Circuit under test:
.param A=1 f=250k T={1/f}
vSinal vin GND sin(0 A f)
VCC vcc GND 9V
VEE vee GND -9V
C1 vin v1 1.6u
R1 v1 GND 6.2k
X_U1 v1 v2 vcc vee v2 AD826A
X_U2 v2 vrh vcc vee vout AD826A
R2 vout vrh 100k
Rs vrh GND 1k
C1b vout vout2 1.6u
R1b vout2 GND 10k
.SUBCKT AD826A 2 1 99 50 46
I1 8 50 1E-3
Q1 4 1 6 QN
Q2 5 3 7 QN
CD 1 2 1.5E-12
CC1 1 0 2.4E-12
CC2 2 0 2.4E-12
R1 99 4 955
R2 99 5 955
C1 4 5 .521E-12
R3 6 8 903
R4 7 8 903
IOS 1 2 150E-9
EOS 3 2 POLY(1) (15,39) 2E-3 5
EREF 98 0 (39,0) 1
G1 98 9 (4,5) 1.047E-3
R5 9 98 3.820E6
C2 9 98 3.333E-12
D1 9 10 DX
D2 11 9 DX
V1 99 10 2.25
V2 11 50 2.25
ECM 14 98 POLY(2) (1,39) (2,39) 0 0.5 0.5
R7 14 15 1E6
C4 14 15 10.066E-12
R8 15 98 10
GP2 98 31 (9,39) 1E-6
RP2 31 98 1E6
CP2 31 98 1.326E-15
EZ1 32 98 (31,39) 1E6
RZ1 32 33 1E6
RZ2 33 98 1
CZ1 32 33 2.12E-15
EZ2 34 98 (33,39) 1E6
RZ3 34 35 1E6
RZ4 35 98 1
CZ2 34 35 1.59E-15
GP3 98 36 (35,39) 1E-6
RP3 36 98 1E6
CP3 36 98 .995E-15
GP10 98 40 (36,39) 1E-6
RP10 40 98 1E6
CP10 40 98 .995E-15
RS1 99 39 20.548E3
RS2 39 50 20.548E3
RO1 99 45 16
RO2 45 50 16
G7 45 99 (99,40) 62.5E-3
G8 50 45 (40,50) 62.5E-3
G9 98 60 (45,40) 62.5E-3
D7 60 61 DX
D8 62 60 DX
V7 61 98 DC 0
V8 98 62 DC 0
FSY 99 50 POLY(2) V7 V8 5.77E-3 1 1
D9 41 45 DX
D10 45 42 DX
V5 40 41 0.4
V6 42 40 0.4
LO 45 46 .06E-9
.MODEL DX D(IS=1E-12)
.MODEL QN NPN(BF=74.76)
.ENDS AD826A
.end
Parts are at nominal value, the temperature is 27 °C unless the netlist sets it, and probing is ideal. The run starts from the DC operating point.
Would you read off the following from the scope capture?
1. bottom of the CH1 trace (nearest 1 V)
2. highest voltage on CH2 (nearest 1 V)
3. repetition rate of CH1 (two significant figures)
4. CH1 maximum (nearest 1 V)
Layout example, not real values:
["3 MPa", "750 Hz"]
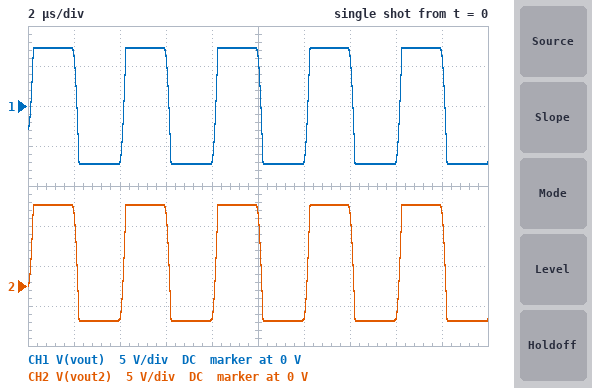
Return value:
["-7 V", "10 V", "250 kHz", "7 V"]
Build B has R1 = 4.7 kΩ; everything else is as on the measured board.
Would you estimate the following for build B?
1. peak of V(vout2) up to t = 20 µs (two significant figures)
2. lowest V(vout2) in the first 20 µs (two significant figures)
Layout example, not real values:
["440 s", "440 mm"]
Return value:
["9.2 V", "-5.4 V"]
